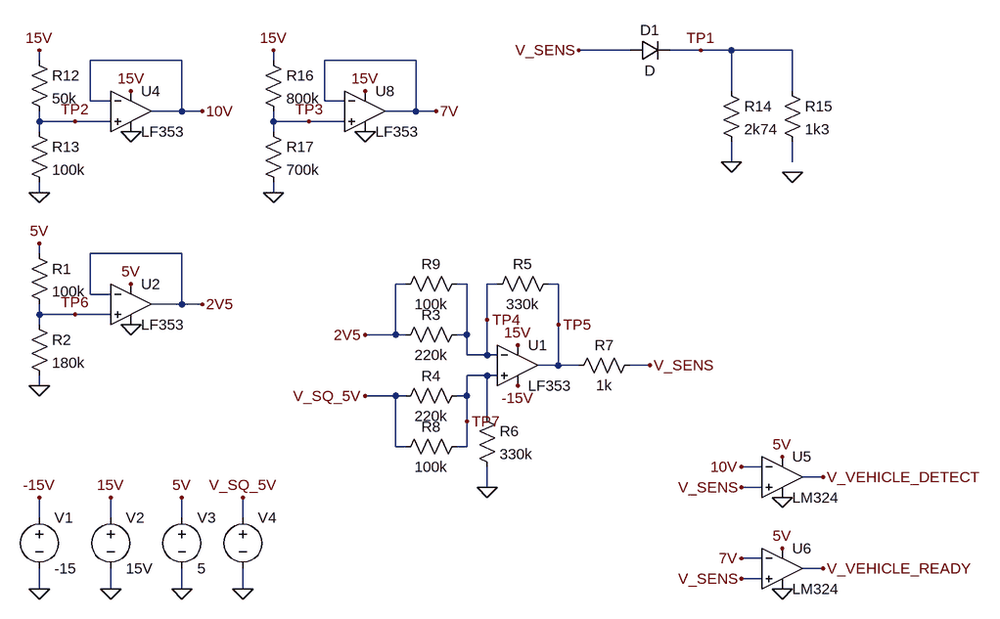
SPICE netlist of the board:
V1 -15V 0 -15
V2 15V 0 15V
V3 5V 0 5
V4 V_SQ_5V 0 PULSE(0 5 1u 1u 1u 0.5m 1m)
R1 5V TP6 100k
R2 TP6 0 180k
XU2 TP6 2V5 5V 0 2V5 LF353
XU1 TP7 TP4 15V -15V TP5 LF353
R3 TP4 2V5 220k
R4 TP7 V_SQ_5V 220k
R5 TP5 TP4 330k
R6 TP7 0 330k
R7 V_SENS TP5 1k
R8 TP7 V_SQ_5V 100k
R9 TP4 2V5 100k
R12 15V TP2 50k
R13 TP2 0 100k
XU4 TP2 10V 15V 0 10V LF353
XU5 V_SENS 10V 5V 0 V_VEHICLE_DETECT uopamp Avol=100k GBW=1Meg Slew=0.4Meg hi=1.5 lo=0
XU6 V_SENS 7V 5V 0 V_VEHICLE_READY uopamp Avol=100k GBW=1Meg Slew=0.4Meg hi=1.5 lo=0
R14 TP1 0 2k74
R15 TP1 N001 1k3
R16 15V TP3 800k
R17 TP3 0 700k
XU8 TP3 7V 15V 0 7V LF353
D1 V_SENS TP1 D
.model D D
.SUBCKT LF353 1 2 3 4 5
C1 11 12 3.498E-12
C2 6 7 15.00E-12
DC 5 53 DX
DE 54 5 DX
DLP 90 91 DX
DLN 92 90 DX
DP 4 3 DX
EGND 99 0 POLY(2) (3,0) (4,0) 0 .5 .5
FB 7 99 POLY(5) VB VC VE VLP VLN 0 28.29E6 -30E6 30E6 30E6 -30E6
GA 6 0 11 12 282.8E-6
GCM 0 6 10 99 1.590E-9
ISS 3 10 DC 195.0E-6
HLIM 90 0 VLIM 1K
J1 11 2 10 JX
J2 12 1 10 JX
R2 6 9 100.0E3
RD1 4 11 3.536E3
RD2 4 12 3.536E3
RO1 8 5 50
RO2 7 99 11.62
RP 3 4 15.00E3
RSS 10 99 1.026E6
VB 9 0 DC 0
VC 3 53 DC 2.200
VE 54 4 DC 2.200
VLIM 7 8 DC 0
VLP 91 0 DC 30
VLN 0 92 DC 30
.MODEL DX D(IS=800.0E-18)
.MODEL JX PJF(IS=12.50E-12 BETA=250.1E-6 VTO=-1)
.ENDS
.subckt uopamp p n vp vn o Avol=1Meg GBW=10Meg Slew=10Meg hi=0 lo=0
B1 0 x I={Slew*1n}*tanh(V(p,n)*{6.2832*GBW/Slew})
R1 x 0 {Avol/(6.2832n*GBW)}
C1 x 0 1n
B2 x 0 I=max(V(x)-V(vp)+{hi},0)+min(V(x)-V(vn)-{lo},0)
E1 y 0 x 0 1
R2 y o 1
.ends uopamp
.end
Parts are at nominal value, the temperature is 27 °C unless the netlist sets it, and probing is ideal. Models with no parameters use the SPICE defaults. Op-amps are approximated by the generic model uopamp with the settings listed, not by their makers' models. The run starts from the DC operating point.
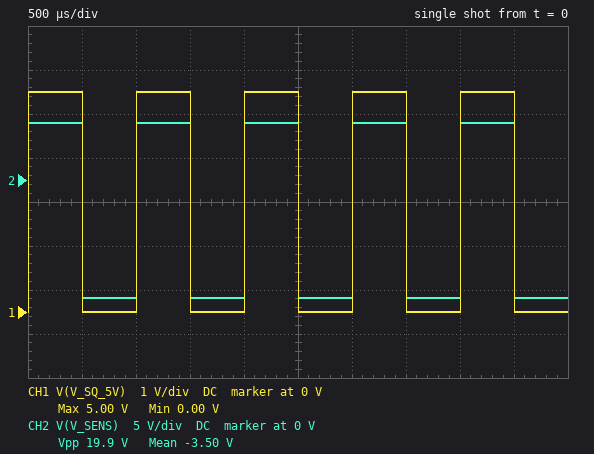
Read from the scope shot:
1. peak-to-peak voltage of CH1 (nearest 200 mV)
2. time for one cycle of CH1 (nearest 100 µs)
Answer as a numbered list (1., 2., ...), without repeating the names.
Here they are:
1. 5.0 V
2. 1.0 ms
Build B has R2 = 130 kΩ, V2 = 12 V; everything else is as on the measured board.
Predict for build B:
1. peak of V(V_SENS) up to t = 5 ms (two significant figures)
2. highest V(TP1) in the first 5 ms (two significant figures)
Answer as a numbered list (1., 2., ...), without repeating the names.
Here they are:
1. 7.8 V
2. 7.1 V
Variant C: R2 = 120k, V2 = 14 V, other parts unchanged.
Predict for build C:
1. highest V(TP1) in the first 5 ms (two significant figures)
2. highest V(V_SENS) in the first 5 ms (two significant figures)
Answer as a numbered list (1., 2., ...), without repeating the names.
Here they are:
1. 7.5 V
2. 8.2 V
